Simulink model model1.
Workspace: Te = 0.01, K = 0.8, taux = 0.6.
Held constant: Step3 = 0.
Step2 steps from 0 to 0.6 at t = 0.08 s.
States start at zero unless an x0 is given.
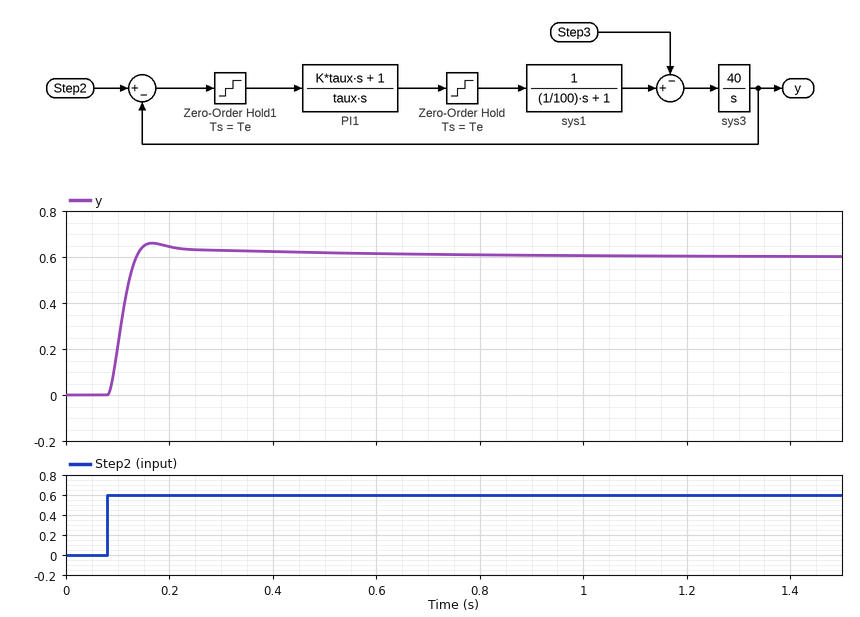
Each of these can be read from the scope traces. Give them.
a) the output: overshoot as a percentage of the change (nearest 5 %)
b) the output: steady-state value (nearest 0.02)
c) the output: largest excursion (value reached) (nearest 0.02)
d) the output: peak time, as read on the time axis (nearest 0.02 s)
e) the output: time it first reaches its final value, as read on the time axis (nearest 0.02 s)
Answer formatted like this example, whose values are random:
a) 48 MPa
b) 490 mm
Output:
a) 10 %
b) 0.60
c) 0.66
d) 0.16 s
e) 0.14 s
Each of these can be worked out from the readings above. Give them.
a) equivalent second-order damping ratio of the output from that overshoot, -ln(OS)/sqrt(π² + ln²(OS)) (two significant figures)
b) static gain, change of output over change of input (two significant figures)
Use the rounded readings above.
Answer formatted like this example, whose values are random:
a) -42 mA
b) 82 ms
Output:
a) 0.59
b) 1.0
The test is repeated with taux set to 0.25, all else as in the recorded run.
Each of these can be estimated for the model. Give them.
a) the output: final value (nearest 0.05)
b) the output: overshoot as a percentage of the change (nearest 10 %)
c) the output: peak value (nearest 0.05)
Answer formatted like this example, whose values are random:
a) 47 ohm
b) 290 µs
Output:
a) 0.60
b) 20 %
c) 0.70
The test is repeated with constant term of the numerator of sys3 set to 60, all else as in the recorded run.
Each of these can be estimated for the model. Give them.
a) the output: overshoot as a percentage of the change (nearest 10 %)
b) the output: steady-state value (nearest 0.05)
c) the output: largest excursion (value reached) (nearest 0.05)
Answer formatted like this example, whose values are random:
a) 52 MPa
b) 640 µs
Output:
a) 20 %
b) 0.60
c) 0.70
